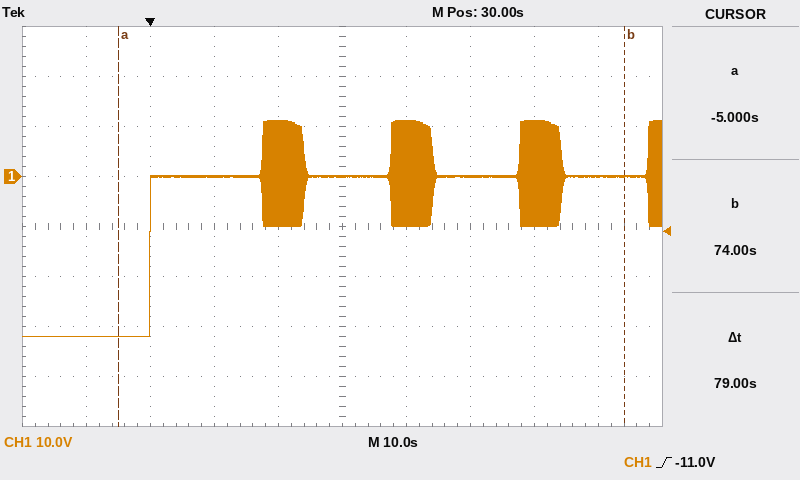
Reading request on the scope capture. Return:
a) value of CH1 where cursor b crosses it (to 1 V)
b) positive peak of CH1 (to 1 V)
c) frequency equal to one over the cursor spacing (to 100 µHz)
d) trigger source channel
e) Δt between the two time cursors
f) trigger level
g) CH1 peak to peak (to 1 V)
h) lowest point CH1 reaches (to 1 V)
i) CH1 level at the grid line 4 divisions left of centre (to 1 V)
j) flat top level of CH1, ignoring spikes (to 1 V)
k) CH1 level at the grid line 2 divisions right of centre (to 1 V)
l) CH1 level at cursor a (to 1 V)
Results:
0 V
11 V
12.7 mHz
CH1
79 s
-11.0 V
43 V
-32 V
-32 V
0 V
0 V
-32 V
